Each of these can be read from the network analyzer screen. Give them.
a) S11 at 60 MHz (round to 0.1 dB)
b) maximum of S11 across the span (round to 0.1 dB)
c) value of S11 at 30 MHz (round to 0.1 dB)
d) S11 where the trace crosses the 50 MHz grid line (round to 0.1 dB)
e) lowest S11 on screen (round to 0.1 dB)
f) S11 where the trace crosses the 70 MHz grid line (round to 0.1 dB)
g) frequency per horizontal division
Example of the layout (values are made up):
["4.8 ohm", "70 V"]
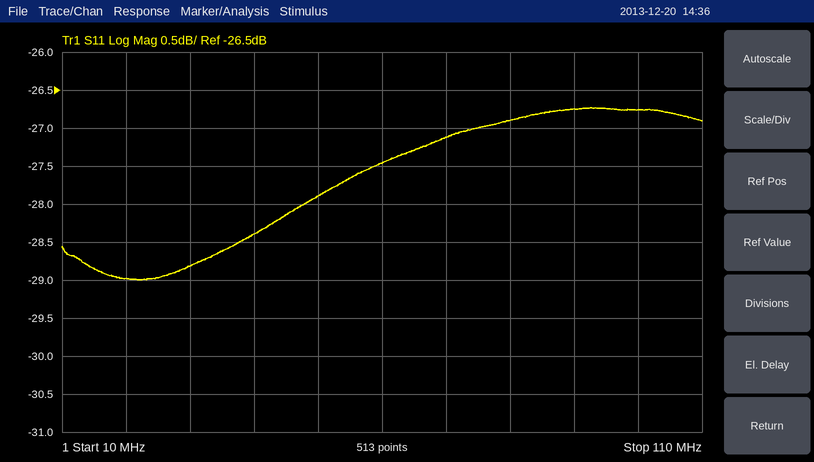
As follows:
["-27.5 dB", "-26.7 dB", "-28.8 dB", "-27.9 dB", "-29.0 dB", "-27.1 dB", "10 MHz"]
